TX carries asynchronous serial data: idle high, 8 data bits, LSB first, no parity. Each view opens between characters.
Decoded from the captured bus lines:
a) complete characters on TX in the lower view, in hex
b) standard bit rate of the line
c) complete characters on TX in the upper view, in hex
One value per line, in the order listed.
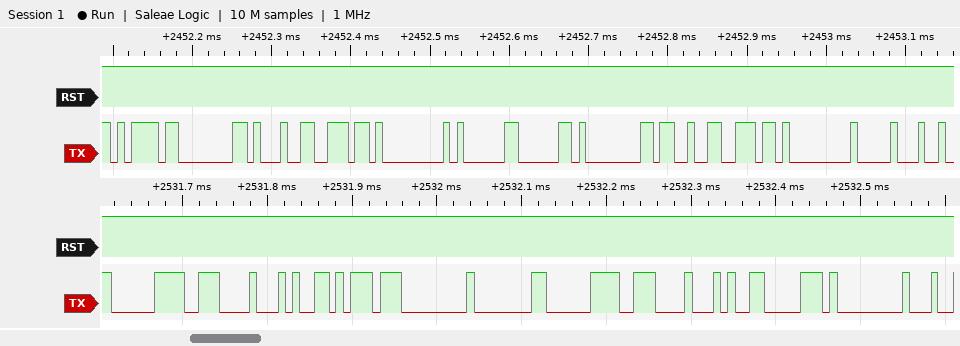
E0, 0E, 94, DD, 00, 80, E0, 0E, 94, 70, 00
115200 baud
BD, 80, 91, 6E, 00, 81, 60, 80, 93, 6E, 00, 10
